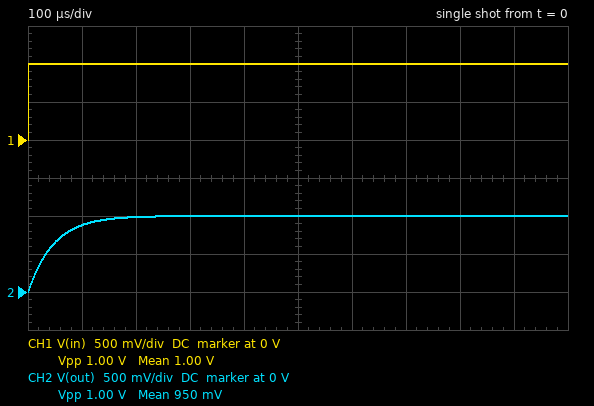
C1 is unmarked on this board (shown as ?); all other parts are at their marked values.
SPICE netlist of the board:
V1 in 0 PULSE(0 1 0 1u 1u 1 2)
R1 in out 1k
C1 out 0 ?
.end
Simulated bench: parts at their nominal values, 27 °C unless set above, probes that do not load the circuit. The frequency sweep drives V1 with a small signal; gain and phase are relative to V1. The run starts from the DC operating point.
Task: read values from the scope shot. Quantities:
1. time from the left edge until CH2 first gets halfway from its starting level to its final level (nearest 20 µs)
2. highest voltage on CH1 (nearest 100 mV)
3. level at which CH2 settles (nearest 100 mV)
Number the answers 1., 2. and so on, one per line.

1. 40 µs
2. 1.0 V
3. 1.0 V
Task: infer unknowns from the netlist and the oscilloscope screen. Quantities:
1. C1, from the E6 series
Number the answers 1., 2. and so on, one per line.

1. 47 nF
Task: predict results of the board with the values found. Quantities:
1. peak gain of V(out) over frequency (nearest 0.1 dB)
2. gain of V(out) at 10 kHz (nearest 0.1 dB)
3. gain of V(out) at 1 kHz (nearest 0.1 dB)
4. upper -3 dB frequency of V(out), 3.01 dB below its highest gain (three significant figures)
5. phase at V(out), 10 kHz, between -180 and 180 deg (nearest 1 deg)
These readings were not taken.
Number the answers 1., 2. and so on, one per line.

1. 0 dB
2. -9.9 dB
3. -0.4 dB
4. 3.39 kHz
5. -71 deg
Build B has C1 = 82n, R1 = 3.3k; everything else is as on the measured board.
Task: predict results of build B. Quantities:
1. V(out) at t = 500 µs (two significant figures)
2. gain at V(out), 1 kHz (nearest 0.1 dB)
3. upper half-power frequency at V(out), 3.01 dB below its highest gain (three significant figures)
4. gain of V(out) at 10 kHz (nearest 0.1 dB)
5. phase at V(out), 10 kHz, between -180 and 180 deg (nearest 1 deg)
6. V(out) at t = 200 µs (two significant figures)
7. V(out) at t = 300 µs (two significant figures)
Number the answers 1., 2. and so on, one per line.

1. 840 mV
2. -5.9 dB
3. 588 Hz
4. -24.6 dB
5. -87 deg
6. 520 mV
7. 670 mV
